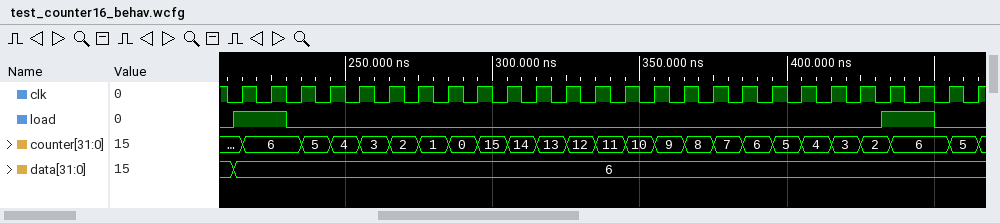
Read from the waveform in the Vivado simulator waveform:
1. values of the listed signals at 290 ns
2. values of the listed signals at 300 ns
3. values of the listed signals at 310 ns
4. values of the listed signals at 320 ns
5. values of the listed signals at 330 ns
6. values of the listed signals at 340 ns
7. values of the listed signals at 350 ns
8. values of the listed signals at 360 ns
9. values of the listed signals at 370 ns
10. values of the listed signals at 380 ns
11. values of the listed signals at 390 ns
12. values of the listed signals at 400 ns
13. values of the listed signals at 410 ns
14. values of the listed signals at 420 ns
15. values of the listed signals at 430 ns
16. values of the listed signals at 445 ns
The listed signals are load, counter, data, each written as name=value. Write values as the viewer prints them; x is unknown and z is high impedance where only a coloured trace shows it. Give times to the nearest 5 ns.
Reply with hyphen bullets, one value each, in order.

- load=0, counter=0, data=6
- load=0, counter=15, data=6
- load=0, counter=14, data=6
- load=0, counter=13, data=6
- load=0, counter=12, data=6
- load=0, counter=11, data=6
- load=0, counter=10, data=6
- load=0, counter=9, data=6
- load=0, counter=8, data=6
- load=0, counter=7, data=6
- load=0, counter=6, data=6
- load=0, counter=5, data=6
- load=0, counter=4, data=6
- load=0, counter=3, data=6
- load=0, counter=2, data=6
- load=1, counter=6, data=6
